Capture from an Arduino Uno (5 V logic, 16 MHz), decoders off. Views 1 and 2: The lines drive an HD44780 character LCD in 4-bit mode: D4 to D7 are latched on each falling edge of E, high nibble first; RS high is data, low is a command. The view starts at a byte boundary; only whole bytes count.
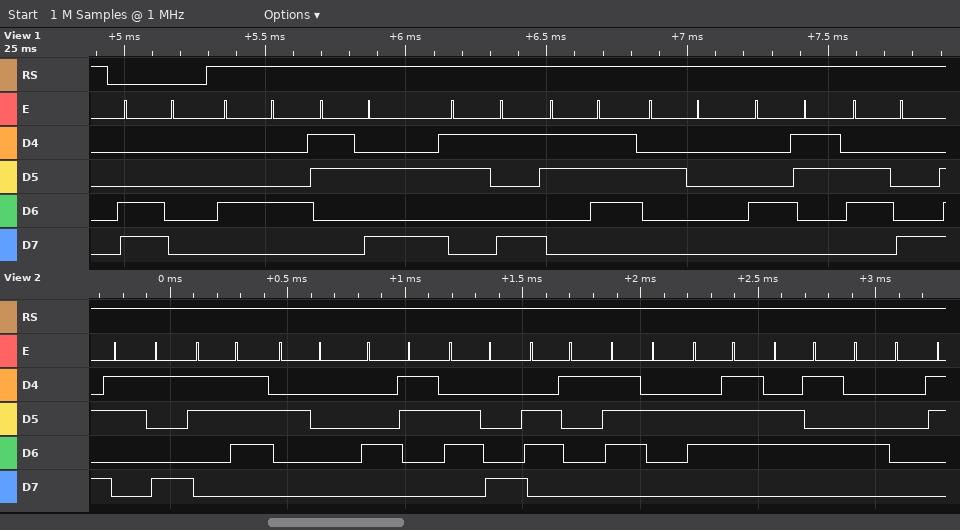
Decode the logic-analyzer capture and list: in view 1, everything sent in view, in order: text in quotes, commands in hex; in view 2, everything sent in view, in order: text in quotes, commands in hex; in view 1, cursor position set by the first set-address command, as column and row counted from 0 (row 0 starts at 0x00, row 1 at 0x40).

0xC0 "D:97 Ch"
"97 Charge@"
column 0, row 1
